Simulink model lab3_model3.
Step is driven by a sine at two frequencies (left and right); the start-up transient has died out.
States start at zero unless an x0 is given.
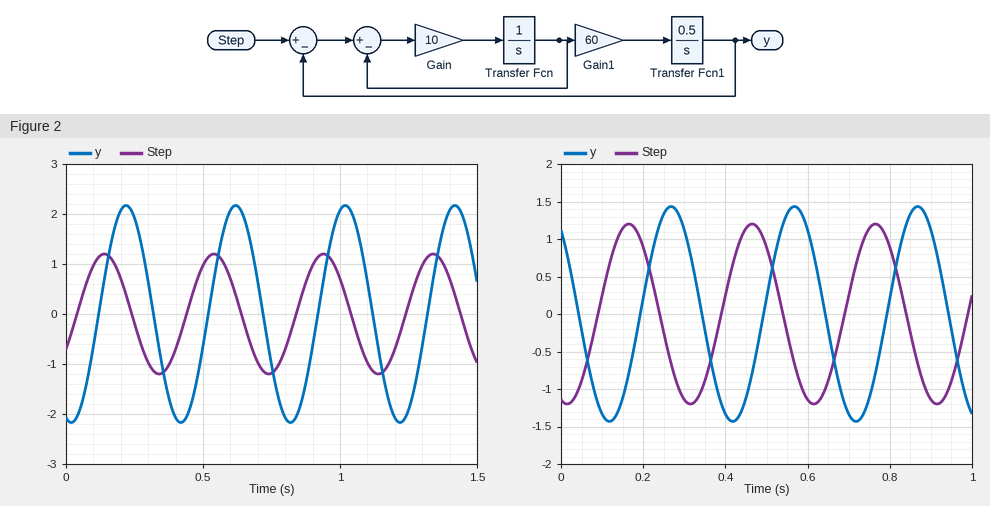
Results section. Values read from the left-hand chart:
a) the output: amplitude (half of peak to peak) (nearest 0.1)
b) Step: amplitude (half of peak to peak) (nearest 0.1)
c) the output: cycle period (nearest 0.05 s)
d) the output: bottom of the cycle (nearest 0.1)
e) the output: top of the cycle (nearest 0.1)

2.2
1.2
0.40 s
-2.2
2.2
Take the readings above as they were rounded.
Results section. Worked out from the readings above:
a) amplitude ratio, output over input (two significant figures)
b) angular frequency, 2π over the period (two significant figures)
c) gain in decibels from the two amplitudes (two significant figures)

1.8
16 rad/s
5.3 dB
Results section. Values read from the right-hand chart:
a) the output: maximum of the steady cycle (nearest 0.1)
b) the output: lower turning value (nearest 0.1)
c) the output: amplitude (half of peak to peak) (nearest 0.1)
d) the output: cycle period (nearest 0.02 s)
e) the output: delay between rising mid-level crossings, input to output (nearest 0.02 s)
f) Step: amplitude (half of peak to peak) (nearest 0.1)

1.4
-1.4
1.4
0.30 s
0.10 s
1.2
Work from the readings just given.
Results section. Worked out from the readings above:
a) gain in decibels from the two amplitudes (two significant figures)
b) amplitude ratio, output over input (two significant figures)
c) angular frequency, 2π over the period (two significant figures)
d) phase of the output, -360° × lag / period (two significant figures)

1.3 dB
1.2
21 rad/s
-120°
